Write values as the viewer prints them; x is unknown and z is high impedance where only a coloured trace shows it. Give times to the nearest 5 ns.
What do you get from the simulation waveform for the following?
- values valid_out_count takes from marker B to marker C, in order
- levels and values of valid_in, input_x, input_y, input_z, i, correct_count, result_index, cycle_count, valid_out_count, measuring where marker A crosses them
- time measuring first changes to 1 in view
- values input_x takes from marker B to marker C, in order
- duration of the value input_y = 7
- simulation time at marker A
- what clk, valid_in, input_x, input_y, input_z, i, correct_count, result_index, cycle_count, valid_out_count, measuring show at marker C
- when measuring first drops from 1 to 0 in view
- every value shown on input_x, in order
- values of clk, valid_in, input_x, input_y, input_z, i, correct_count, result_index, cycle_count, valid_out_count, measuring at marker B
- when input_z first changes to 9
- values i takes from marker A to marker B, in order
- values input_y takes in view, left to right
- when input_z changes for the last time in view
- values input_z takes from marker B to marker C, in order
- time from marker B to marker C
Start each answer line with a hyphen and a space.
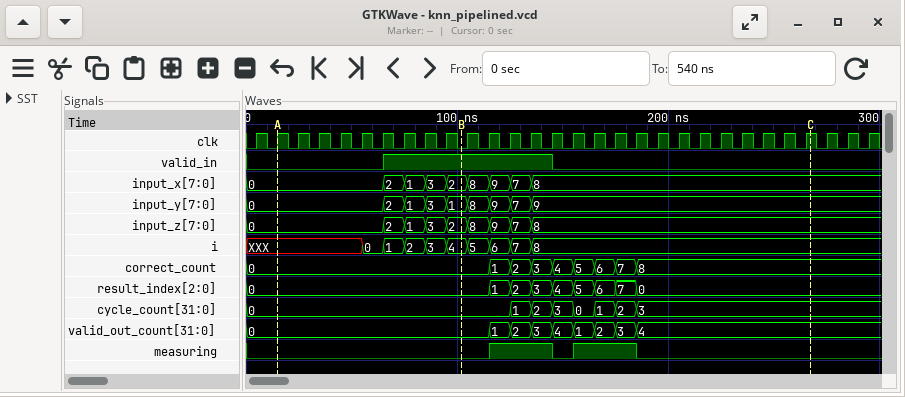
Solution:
- 0, 1, 2, 3, 4, 1, 2, 3, 4
- valid_in=0, input_x=0, input_y=0, input_z=0, i=XXX, correct_count=0, result_index=0, cycle_count=0, valid_out_count=0, measuring=0
- 115 ns
- 2, 8, 9, 7, 8
- 10 ns
- 15 ns
- clk=1, valid_in=0, input_x=8, input_y=9, input_z=8, i=8, correct_count=8, result_index=0, cycle_count=3, valid_out_count=4, measuring=0
- 145 ns
- 0, 2, 1, 3, 2, 8, 9, 7, 8
- clk=0, valid_in=1, input_x=2, input_y=1, input_z=2, i=4, correct_count=0, result_index=0, cycle_count=0, valid_out_count=0, measuring=0
- 115 ns
- XXX, 0, 1, 2, 3, 4
- 0, 2, 1, 3, 1, 8, 9, 7, 9
- 135 ns
- 2, 8, 9, 7, 8
- 165 ns
